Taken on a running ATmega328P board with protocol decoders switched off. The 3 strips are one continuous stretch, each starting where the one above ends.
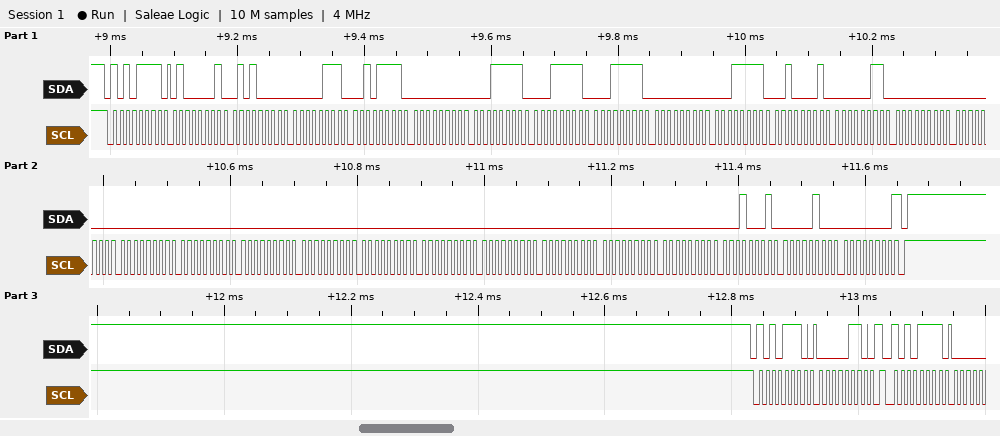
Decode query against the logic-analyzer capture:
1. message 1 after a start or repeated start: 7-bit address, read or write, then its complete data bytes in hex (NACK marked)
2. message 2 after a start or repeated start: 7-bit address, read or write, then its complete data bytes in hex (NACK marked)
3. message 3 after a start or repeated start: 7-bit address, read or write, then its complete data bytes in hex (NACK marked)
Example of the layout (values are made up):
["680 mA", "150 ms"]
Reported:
["0x57 read: 41 50 07 2F 00 1F 1F 1F 00 1F 21 03 00 00 00 00 00 00 00 00 00 00 00 00 11 04 00 NACK", "0x57 write: 06", "0x57 read"]
